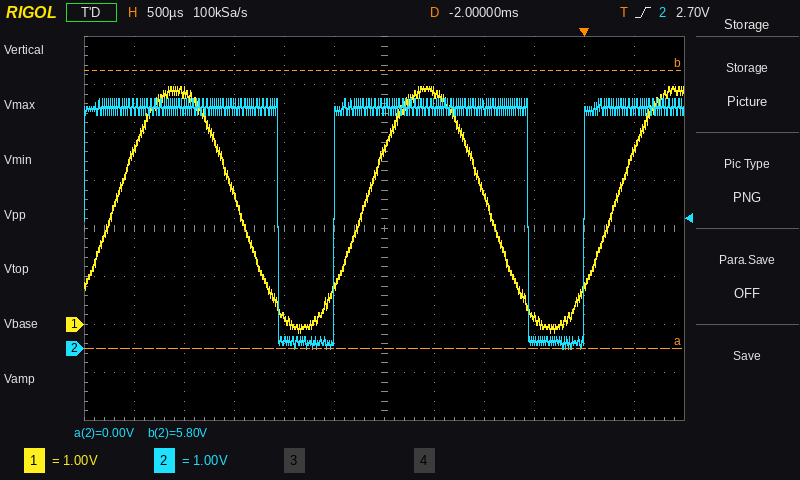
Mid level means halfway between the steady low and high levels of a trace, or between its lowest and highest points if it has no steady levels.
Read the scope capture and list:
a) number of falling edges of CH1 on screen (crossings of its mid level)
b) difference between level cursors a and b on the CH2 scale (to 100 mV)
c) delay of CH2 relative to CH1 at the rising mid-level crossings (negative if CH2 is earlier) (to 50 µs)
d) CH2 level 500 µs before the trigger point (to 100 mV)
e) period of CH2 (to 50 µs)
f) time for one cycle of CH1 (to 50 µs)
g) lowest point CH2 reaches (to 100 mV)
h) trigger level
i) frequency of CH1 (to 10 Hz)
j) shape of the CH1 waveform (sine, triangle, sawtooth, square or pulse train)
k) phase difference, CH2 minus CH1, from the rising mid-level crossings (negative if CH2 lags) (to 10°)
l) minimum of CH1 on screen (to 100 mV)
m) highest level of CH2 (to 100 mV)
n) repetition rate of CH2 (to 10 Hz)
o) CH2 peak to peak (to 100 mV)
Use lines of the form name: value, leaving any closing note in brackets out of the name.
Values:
number of falling edges of CH1 on screen: 2
difference between level cursors a and b on the CH2 scale: 5.8 V
delay of CH2 relative to CH1 at the rising mid-level crossings (negative if CH2 is earlier): -300 µs
CH2 level 500 µs before the trigger point: 200 mV
period of CH2: 2.50 ms
time for one cycle of CH1: 2.50 ms
lowest point CH2 reaches: 0.0 V
trigger level: 2.70 V
frequency of CH1: 400 Hz
shape of the CH1 waveform: sine
phase difference, CH2 minus CH1, from the rising mid-level crossings (negative if CH2 lags): +40°
minimum of CH1 on screen: -200 mV
highest level of CH2: 5.2 V
repetition rate of CH2: 400 Hz
CH2 peak to peak: 5.2 V
